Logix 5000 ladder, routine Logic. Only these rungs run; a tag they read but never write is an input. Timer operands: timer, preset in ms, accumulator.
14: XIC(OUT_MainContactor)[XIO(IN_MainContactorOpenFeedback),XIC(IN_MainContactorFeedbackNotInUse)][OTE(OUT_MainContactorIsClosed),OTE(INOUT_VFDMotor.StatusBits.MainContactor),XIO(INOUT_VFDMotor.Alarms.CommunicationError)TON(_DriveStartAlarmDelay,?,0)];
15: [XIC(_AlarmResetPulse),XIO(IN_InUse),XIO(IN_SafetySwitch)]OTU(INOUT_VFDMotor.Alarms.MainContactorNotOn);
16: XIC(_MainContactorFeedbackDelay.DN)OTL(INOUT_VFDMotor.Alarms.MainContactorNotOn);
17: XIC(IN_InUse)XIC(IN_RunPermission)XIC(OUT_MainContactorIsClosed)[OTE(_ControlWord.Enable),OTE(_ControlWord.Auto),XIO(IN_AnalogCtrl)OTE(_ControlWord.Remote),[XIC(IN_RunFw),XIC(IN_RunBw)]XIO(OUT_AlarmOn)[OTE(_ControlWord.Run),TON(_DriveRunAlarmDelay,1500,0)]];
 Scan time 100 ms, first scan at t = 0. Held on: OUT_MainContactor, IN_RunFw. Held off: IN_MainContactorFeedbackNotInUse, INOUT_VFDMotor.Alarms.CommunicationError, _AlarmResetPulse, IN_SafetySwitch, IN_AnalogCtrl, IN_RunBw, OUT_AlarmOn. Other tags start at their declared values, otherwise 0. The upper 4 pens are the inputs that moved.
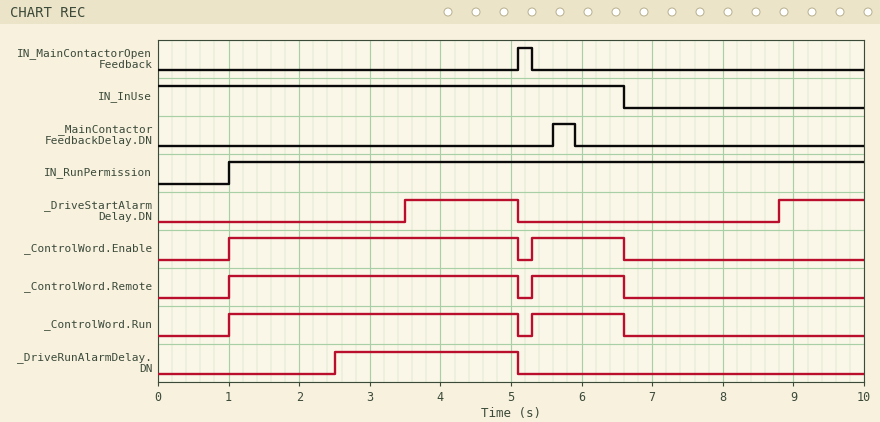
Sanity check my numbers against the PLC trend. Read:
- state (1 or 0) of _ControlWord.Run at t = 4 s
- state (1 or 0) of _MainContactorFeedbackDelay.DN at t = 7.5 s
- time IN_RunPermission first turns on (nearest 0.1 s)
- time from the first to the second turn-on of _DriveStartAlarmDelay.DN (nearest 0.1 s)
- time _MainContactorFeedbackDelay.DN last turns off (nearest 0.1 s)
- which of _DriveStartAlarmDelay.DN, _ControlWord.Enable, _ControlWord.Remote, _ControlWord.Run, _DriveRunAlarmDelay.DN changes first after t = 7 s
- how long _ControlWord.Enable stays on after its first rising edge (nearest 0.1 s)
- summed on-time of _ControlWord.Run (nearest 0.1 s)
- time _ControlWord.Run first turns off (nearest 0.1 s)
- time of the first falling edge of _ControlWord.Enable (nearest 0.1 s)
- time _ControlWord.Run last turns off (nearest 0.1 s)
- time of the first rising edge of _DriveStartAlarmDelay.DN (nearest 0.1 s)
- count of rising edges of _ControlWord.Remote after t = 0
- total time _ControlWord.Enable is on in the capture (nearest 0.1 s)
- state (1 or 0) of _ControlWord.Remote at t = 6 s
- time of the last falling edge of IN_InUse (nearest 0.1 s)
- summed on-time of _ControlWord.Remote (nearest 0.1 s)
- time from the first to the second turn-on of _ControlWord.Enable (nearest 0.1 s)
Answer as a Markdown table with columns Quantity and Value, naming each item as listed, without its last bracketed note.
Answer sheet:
| Quantity | Value |
|---|---|
| state (1 or 0) of _ControlWord.Run at t = 4 s | 1 |
| state (1 or 0) of _MainContactorFeedbackDelay.DN at t = 7.5 s | 0 |
| time IN_RunPermission first turns on | 1.0 s |
| time from the first to the second turn-on of _DriveStartAlarmDelay.DN | 5.3 s |
| time _MainContactorFeedbackDelay.DN last turns off | 5.9 s |
| which of _DriveStartAlarmDelay.DN, _ControlWord.Enable, _ControlWord.Remote, _ControlWord.Run, _DriveRunAlarmDelay.DN changes first after t = 7 s | _DriveStartAlarmDelay.DN |
| how long _ControlWord.Enable stays on after its first rising edge | 4.1 s |
| summed on-time of _ControlWord.Run | 5.4 s |
| time _ControlWord.Run first turns off | 5.1 s |
| time of the first falling edge of _ControlWord.Enable | 5.1 s |
| time _ControlWord.Run last turns off | 6.6 s |
| time of the first rising edge of _DriveStartAlarmDelay.DN | 3.5 s |
| count of rising edges of _ControlWord.Remote after t = 0 | 2 |
| total time _ControlWord.Enable is on in the capture | 5.4 s |
| state (1 or 0) of _ControlWord.Remote at t = 6 s | 1 |
| time of the last falling edge of IN_InUse | 6.6 s |
| summed on-time of _ControlWord.Remote | 5.4 s |
| time from the first to the second turn-on of _ControlWord.Enable | 4.3 s |
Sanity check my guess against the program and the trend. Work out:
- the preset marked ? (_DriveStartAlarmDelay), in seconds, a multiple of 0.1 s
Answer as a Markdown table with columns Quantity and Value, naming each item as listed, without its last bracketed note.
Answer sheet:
| Quantity | Value |
|---|---|
| the preset marked ? (_DriveStartAlarmDelay), in seconds, a multiple of 0.1 s | 3.5 s |
